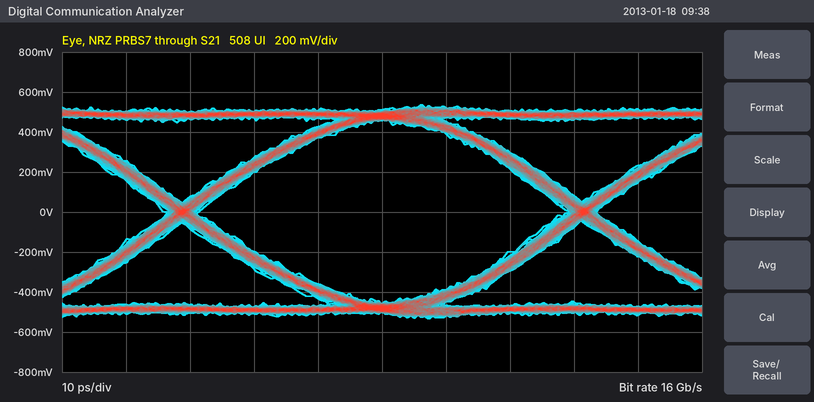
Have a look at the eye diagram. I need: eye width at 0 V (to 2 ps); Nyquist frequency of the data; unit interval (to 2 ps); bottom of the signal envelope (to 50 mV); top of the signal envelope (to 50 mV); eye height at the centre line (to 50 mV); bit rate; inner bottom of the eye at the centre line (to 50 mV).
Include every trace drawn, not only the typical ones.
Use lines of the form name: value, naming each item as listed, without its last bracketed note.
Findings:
eye width at 0 V: 58 ps
Nyquist frequency of the data: 8 GHz
unit interval: 62 ps
bottom of the signal envelope: -550 mV
top of the signal envelope: 550 mV
eye height at the centre line: 900 mV
bit rate: 16 Gb/s
inner bottom of the eye at the centre line: -450 mV
